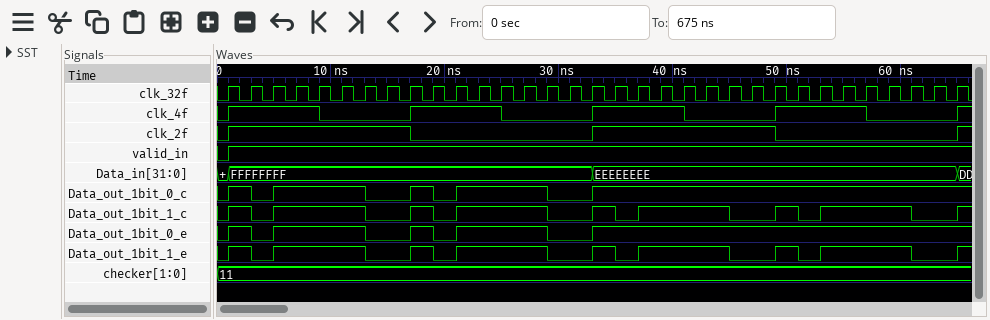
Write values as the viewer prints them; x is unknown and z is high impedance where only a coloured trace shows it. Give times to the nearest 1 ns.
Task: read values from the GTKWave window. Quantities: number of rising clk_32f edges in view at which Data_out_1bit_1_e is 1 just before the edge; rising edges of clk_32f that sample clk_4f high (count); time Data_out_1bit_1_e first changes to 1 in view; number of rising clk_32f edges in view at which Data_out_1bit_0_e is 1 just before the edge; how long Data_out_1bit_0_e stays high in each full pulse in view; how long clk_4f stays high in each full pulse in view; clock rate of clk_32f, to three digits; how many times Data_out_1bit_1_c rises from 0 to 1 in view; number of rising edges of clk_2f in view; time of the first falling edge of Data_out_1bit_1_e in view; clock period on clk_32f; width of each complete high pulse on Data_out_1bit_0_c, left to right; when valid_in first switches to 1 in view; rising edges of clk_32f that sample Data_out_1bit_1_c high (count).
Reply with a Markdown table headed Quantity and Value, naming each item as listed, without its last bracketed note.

| Quantity | Value |
|---|---|
| number of rising clk_32f edges in view at which Data_out_1bit_1_e is 1 just before the edge | 20 |
| rising edges of clk_32f that sample clk_4f high | 16 |
| time Data_out_1bit_1_e first changes to 1 in view | 1 ns |
| number of rising clk_32f edges in view at which Data_out_1bit_0_e is 1 just before the edge | 26 |
| how long Data_out_1bit_0_e stays high in each full pulse in view | 2 ns, 8 ns, 2 ns, 8 ns |
| how long clk_4f stays high in each full pulse in view | 8 ns, 8 ns, 8 ns, 8 ns |
| clock rate of clk_32f, to three digits | 500 MHz |
| how many times Data_out_1bit_1_c rises from 0 to 1 in view | 9 |
| number of rising edges of clk_2f in view | 3 |
| time of the first falling edge of Data_out_1bit_1_e in view | 3 ns |
| clock period on clk_32f | 2 ns |
| width of each complete high pulse on Data_out_1bit_0_c, left to right | 2 ns, 8 ns, 2 ns, 8 ns |
| when valid_in first switches to 1 in view | 1 ns |
| rising edges of clk_32f that sample Data_out_1bit_1_c high | 20 |
